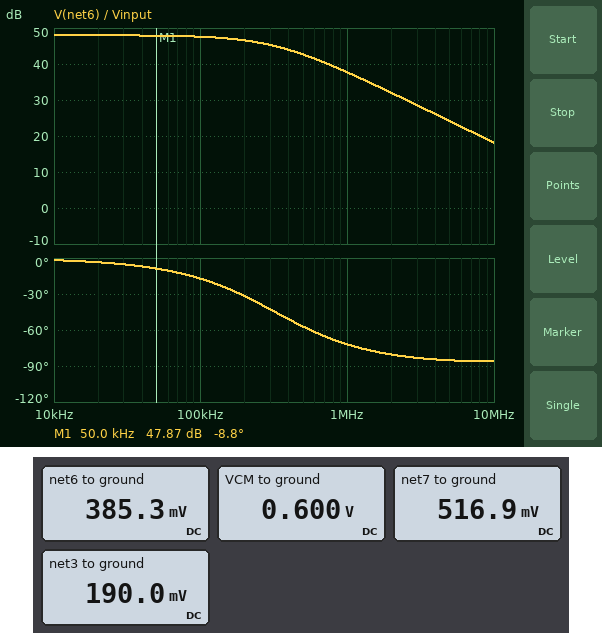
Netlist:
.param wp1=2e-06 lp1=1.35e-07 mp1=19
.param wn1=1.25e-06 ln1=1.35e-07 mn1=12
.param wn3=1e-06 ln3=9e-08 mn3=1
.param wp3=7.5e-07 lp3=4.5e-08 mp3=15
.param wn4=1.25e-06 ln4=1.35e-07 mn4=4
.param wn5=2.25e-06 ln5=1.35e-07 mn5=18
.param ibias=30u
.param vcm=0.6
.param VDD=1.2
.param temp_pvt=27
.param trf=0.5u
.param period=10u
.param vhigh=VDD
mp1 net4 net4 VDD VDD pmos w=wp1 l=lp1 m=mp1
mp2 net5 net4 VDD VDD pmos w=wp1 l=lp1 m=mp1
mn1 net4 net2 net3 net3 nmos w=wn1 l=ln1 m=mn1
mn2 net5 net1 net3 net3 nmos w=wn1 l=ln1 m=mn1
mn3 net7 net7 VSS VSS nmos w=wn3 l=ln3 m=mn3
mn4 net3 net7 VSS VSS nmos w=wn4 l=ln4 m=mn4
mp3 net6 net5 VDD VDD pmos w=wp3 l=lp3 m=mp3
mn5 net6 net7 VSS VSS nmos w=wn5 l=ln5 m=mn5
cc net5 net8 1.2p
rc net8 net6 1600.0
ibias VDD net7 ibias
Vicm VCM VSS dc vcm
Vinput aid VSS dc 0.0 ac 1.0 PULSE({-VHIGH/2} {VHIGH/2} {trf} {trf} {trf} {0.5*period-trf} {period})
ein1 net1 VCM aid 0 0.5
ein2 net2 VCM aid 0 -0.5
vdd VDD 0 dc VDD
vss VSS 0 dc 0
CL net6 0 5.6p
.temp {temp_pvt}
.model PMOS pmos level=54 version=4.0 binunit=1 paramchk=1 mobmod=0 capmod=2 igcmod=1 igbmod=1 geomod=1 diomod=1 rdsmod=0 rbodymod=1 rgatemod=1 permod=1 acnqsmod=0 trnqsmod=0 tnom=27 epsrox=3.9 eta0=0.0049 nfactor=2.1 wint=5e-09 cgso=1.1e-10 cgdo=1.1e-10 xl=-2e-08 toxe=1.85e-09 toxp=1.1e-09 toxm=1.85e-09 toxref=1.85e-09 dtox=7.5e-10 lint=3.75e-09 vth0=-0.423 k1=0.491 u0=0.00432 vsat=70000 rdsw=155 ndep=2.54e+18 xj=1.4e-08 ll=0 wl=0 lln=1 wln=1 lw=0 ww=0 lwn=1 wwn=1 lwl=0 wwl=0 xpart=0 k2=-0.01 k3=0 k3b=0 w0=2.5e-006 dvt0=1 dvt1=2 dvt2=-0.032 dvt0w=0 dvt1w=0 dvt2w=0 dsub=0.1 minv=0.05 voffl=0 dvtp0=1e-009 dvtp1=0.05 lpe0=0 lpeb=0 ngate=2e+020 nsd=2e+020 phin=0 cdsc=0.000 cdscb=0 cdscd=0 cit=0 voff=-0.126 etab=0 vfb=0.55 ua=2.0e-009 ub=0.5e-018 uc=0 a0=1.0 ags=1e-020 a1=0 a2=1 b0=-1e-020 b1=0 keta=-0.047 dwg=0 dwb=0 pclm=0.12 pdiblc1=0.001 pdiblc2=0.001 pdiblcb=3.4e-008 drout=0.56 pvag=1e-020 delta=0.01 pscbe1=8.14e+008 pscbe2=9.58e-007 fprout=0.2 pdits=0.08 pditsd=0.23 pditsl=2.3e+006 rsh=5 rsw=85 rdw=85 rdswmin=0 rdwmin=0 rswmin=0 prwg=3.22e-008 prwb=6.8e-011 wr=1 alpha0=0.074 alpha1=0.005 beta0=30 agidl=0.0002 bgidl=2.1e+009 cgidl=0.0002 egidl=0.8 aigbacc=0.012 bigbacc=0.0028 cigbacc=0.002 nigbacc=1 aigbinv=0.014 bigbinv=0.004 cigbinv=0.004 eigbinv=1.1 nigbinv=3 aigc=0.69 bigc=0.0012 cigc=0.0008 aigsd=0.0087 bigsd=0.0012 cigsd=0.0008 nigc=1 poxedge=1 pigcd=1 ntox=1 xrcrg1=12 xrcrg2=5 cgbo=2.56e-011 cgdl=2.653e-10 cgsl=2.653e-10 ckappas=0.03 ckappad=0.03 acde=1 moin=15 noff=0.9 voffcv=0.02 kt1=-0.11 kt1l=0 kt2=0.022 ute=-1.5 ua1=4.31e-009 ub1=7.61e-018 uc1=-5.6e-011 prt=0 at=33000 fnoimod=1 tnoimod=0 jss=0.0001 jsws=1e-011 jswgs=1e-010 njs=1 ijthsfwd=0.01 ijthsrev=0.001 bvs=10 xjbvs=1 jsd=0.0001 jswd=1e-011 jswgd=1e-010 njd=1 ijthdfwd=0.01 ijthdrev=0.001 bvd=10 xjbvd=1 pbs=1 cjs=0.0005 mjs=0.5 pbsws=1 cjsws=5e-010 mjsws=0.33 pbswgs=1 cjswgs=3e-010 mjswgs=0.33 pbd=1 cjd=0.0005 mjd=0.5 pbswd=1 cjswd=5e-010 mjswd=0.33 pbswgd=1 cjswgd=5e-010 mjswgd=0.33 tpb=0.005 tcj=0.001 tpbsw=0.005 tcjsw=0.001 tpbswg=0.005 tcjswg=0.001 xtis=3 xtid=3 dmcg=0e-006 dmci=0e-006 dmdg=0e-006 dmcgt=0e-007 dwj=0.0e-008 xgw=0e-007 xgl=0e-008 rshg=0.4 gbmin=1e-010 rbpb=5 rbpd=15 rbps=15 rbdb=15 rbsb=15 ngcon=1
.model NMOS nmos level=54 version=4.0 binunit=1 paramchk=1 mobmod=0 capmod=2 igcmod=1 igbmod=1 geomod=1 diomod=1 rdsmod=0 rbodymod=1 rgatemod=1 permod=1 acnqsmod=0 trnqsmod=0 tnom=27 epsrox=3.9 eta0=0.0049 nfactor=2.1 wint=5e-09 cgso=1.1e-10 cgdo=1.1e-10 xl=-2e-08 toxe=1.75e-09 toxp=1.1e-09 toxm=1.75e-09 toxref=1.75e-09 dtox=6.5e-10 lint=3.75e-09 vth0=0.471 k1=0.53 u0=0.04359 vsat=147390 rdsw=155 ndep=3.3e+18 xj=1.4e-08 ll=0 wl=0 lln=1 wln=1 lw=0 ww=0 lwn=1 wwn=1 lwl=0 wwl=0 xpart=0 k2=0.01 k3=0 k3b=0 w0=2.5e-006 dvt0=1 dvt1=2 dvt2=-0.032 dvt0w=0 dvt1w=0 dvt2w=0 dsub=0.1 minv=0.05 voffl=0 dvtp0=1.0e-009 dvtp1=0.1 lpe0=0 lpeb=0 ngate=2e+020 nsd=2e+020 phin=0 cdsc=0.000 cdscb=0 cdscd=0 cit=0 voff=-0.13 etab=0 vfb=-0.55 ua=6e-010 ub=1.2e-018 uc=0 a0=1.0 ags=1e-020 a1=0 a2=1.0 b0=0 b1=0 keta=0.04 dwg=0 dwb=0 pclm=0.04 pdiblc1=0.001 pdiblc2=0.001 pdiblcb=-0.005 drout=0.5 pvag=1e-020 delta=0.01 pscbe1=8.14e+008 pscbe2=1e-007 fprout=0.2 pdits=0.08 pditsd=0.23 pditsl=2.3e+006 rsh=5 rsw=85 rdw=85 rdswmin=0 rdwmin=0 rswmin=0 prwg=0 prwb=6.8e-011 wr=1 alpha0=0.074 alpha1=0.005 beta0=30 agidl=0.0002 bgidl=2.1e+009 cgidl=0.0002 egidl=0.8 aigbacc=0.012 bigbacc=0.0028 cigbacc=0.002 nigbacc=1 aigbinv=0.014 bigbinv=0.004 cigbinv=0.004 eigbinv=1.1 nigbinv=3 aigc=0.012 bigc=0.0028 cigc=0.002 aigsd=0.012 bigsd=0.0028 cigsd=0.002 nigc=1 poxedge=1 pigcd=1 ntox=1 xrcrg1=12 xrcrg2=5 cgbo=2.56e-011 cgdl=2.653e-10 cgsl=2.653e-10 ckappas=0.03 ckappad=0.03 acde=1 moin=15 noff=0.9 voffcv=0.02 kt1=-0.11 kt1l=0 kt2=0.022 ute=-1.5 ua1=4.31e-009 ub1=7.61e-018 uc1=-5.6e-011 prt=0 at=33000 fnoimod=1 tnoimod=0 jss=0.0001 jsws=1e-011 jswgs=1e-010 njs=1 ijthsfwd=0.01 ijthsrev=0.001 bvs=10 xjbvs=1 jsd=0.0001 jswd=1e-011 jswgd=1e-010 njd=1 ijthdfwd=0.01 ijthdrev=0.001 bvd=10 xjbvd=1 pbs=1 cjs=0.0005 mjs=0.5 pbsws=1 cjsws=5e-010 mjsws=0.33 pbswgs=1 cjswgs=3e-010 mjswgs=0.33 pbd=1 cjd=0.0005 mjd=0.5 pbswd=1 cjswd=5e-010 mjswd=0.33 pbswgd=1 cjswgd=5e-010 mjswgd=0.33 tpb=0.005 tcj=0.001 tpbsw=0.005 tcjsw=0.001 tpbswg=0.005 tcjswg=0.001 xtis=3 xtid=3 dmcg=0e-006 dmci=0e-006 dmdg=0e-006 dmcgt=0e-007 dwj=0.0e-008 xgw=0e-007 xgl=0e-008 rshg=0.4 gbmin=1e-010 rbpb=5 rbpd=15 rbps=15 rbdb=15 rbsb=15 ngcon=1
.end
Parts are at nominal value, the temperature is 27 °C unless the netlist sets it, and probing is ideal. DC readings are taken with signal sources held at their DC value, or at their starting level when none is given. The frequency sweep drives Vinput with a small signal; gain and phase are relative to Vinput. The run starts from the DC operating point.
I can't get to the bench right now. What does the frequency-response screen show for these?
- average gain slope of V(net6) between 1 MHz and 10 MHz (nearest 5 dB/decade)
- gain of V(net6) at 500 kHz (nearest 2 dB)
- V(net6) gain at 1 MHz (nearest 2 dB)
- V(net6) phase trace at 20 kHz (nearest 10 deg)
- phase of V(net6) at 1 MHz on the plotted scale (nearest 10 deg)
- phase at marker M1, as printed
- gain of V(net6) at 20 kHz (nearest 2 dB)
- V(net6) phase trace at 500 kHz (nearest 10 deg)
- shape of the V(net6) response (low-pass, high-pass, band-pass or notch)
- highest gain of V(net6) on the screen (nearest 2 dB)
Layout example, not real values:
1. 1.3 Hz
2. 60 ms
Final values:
1. -20 dB/decade
2. 42 dB
3. 38 dB
4. 0 deg
5. -70 deg
6. -8.8 deg
7. 48 dB
8. -60 deg
9. low-pass
10. 48 dB
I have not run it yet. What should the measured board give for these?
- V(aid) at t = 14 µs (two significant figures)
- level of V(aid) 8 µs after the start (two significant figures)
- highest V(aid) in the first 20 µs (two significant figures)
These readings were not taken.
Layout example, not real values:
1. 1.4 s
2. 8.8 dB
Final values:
1. 600 mV
2. -600 mV
3. 600 mV
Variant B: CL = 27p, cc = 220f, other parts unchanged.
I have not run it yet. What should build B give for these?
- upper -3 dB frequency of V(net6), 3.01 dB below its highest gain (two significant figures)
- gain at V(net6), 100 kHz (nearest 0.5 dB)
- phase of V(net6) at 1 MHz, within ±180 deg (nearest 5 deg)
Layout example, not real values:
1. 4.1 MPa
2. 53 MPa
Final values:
1. 1.4 MHz
2. 48.0 dB
3. -35 deg
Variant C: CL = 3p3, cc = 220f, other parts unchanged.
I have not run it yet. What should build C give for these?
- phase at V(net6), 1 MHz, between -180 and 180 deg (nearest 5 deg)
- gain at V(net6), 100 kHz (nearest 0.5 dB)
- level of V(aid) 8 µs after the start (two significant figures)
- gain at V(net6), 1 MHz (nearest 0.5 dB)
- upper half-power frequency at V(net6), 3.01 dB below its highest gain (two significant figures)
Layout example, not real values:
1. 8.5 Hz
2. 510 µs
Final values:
1. -30 deg
2. 48.0 dB
3. -600 mV
4. 46.5 dB
5. 1.6 MHz
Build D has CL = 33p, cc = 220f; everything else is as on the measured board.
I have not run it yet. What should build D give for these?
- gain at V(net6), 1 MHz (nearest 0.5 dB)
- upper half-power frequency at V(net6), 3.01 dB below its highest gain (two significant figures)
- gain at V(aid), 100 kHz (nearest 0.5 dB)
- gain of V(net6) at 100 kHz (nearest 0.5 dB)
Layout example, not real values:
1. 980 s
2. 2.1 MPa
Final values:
1. 46.0 dB
2. 1.4 MHz
3. 0 dB
4. 48.0 dB
